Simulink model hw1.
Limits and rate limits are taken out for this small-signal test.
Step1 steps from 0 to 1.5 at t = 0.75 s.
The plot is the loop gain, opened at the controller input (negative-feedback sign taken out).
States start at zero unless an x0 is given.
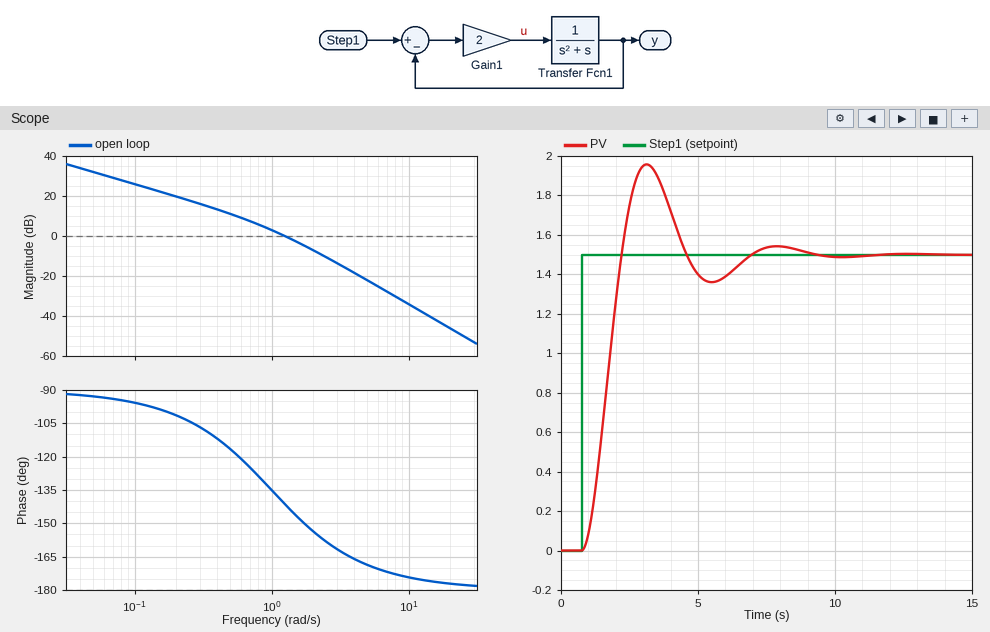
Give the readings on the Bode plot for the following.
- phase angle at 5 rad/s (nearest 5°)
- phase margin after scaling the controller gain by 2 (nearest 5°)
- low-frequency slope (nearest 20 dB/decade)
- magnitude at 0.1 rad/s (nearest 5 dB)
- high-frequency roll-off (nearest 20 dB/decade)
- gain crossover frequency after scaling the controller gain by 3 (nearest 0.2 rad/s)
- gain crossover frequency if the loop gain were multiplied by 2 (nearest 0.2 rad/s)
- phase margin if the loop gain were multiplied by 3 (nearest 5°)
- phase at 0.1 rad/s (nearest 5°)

-170°
30°
-20 dB/decade
25 dB
-40 dB/decade
2.4 rad/s
1.8 rad/s
25°
-95°
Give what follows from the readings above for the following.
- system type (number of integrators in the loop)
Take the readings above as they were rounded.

1
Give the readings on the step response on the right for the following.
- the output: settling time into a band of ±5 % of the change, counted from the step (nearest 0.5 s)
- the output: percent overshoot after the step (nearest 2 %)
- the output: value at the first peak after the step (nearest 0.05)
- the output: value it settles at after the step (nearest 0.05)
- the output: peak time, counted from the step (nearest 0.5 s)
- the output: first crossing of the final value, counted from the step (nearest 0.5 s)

5.5 s
30 %
1.95
1.50
2.5 s
1.5 s
